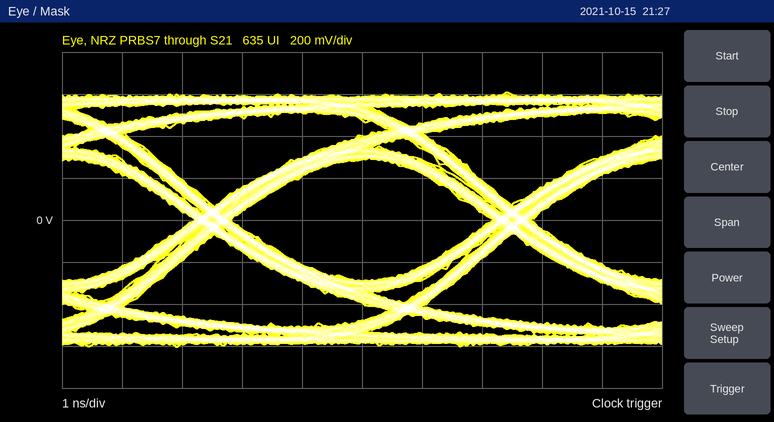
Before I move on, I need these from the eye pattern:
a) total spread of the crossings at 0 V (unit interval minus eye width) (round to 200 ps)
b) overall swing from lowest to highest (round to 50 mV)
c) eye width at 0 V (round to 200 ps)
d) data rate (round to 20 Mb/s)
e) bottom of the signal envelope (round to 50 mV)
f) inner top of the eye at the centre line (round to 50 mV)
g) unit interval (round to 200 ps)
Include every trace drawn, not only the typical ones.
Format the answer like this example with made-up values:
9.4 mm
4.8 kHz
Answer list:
600 ps
1.20 V
4.4 ns
200 Mb/s
-600 mV
300 mV
5.0 ns
